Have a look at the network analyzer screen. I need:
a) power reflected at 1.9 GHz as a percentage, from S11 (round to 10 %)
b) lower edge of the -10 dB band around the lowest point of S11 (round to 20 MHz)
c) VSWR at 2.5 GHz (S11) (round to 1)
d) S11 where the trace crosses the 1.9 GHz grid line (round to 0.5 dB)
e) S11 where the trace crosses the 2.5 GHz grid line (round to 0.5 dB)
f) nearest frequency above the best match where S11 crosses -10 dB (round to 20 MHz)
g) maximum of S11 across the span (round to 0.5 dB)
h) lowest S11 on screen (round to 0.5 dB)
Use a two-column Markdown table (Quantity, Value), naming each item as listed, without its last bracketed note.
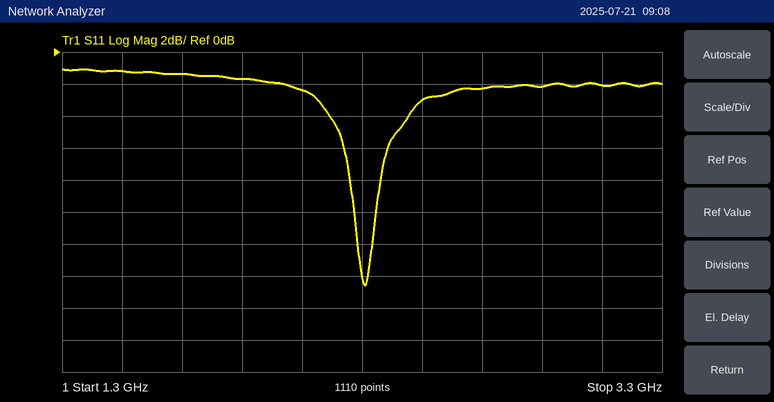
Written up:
| Quantity | Value |
|---|---|
| power reflected at 1.9 GHz as a percentage, from S11 | 70 % |
| lower edge of the -10 dB band around the lowest point of S11 | 2.28 GHz |
| VSWR at 2.5 GHz (S11) | 6 |
| S11 where the trace crosses the 1.9 GHz grid line | -1.5 dB |
| S11 where the trace crosses the 2.5 GHz grid line | -3.0 dB |
| nearest frequency above the best match where S11 crosses -10 dB | 2.34 GHz |
| maximum of S11 across the span | -1.0 dB |
| lowest S11 on screen | -14.5 dB |
